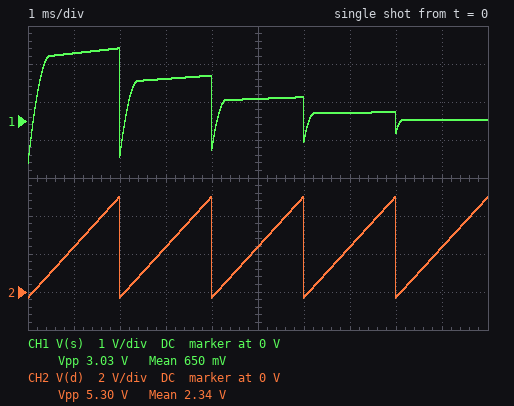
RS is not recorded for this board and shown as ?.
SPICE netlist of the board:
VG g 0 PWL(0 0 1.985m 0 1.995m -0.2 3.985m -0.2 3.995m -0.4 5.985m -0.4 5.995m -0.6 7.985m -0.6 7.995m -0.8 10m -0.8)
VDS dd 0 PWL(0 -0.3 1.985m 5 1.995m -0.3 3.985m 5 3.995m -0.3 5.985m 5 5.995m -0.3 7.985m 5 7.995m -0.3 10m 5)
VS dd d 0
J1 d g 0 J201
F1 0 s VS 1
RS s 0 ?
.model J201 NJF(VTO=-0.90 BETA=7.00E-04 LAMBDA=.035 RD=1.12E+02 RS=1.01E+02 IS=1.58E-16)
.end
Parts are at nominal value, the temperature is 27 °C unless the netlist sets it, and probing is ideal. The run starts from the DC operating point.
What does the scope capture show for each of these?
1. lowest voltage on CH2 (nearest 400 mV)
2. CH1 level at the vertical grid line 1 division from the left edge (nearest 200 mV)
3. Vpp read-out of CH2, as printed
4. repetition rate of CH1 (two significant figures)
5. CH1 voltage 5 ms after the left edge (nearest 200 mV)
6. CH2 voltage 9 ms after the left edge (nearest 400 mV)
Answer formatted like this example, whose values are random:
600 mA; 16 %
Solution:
-400 mV; 1.8 V; 5.30 V; 490 Hz; 600 mV; 2.4 V
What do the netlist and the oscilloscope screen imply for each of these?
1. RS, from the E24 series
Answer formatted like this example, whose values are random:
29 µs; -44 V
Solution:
3.3 kΩ
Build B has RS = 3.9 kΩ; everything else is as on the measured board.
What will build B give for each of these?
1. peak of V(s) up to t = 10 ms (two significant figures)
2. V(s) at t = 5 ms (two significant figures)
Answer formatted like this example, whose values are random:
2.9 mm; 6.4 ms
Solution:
2.3 V; 690 mV
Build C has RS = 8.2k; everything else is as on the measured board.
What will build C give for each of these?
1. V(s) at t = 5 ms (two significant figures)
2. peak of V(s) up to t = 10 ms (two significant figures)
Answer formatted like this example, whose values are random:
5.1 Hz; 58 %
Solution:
1.4 V; 4.8 V
